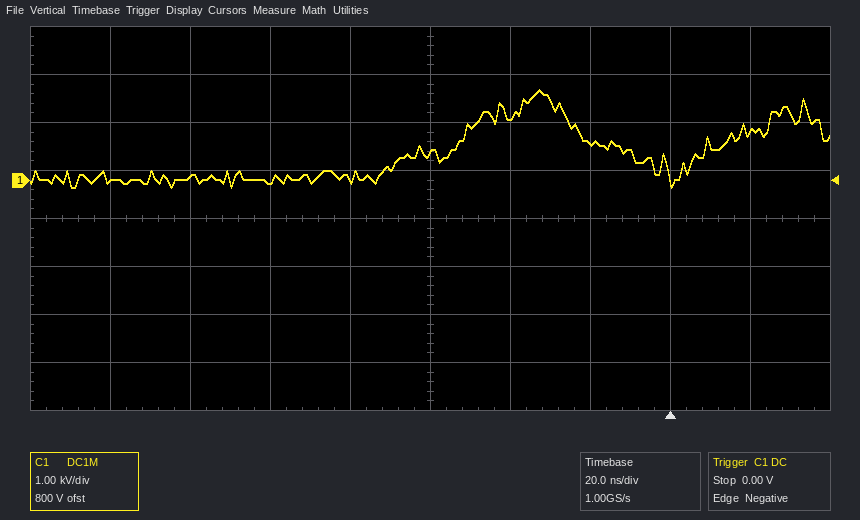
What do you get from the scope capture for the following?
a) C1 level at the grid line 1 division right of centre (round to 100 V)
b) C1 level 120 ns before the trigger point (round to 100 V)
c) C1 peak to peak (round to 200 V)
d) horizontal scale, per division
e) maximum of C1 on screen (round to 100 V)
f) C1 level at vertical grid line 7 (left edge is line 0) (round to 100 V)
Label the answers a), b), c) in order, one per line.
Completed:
a) 1.3 kV
b) 100 V
c) 2.0 kV
d) 20 ns
e) 1.9 kV
f) 800 V
